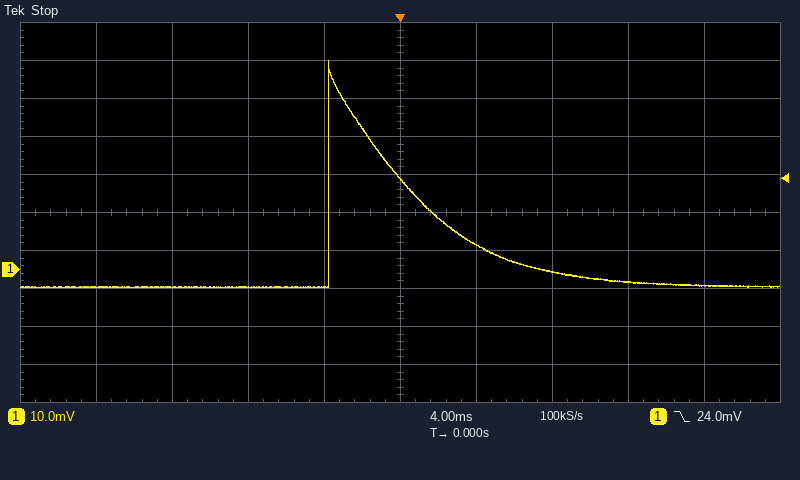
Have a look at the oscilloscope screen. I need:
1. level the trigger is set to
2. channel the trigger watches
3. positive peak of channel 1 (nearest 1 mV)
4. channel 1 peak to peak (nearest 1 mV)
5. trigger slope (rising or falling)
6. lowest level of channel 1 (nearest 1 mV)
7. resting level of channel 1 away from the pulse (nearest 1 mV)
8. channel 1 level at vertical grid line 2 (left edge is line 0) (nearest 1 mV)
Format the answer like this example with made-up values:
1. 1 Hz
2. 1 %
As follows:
1. 24.0 mV
2. channel 1
3. 55 mV
4. 60 mV
5. falling
6. -5 mV
7. -5 mV
8. -5 mV
